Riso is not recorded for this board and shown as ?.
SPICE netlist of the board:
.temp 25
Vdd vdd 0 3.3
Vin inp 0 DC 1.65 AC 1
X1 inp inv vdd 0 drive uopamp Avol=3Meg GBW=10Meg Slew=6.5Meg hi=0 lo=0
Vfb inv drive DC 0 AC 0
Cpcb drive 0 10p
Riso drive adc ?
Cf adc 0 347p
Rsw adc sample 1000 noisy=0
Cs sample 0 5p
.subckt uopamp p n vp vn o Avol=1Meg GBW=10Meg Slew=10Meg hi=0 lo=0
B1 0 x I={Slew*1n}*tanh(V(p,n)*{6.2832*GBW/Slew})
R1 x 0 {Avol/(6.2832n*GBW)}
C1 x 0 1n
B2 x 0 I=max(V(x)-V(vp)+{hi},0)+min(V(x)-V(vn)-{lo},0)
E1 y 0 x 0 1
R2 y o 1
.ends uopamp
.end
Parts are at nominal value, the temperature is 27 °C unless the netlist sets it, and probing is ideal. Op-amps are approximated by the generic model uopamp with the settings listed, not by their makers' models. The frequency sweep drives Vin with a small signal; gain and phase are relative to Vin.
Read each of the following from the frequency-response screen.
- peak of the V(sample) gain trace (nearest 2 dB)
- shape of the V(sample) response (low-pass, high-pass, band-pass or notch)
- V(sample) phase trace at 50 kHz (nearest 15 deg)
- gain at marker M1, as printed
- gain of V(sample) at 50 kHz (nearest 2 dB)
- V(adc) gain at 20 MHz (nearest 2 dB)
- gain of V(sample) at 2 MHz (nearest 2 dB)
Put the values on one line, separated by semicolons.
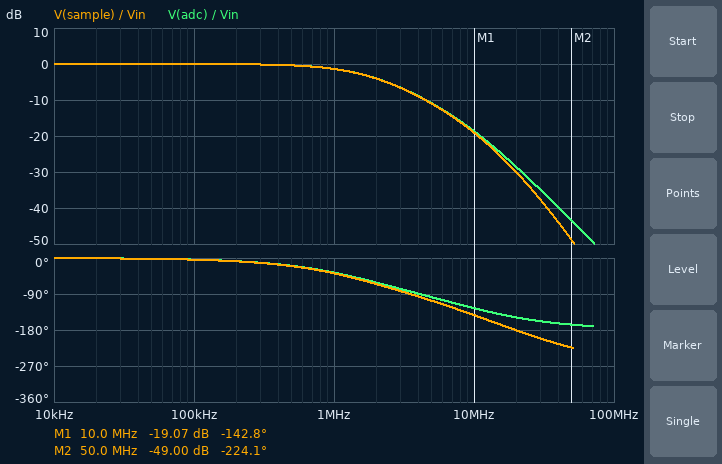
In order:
0 dB; low-pass; 0 deg; -19.07 dB; 0 dB; -28 dB; -4 dB
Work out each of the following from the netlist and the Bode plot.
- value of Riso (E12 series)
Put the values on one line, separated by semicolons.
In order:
270 Ω
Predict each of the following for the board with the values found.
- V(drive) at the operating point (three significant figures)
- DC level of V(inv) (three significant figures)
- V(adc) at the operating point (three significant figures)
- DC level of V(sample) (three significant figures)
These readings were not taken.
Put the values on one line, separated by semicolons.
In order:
1.65 V; 1.65 V; 1.65 V; 1.65 V
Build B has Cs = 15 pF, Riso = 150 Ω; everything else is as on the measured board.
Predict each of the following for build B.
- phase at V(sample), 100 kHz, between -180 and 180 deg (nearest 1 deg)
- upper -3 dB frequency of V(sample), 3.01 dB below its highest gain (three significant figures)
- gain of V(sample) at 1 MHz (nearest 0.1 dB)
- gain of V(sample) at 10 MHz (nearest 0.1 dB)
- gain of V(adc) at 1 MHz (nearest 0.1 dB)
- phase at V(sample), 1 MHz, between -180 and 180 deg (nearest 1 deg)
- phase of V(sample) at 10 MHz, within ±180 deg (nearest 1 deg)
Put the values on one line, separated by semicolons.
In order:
-3 deg; 2.56 MHz; -0.6 dB; -16.7 dB; -0.5 dB; -30 deg; -161 deg
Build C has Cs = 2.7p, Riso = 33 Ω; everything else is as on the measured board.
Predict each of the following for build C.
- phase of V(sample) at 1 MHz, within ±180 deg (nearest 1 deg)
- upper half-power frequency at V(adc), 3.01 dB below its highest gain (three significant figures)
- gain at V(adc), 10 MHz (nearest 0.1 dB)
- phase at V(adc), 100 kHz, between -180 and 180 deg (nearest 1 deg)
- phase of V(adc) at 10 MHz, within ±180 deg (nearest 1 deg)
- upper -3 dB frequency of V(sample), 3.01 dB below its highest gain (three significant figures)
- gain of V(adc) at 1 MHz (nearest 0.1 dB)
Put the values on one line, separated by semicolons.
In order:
-11 deg; 7.47 MHz; -4.8 dB; -1 deg; -82 deg; 7.37 MHz; -0.1 dB
